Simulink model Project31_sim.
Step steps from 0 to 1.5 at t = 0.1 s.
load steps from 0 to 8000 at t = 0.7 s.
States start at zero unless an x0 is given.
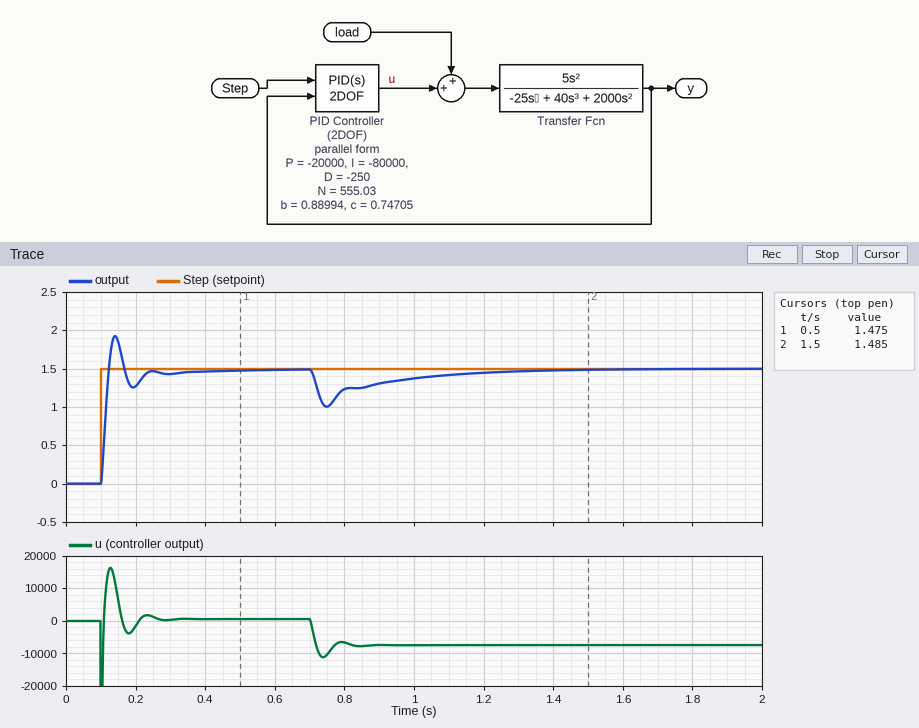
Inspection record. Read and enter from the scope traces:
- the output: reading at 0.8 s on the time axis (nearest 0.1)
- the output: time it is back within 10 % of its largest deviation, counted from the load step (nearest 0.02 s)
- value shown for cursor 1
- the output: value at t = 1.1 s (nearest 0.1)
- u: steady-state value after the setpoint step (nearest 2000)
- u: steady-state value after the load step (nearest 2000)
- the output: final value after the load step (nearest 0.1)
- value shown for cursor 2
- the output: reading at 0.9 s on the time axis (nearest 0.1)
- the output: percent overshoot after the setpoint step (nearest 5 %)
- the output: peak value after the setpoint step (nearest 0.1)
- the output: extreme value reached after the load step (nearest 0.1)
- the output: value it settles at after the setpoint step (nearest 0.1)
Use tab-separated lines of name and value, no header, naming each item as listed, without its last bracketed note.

the output: reading at 0.8 s on the time axis	1.2
the output: time it is back within 10 % of its largest deviation, counted from the load step	0.52 s
value shown for cursor 1	1.475
the output: value at t = 1.1 s	1.4
u: steady-state value after the setpoint step	0
u: steady-state value after the load step	-8000
the output: final value after the load step	1.5
value shown for cursor 2	1.485
the output: reading at 0.9 s on the time axis	1.3
the output: percent overshoot after the setpoint step	30 %
the output: peak value after the setpoint step	1.9
the output: extreme value reached after the load step	1.0
the output: value it settles at after the setpoint step	1.5
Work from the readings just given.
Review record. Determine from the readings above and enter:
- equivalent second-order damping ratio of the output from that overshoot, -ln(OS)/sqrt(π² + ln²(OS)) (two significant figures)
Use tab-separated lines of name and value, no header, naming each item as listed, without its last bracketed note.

equivalent second-order damping ratio of the output from that overshoot, -ln(OS)/sqrt(π² + ln²(OS))	0.36
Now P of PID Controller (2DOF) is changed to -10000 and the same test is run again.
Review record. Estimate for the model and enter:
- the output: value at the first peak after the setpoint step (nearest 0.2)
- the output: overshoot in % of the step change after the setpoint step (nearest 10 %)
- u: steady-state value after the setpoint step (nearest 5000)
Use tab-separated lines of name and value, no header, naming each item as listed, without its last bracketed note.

the output: value at the first peak after the setpoint step	1.8
the output: overshoot in % of the step change after the setpoint step	20 %
u: steady-state value after the setpoint step	0
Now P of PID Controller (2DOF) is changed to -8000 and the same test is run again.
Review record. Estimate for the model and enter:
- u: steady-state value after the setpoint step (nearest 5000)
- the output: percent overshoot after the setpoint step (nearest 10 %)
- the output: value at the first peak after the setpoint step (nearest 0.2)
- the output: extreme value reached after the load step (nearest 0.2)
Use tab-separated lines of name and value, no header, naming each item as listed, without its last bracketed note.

u: steady-state value after the setpoint step	0
the output: percent overshoot after the setpoint step	20 %
the output: value at the first peak after the setpoint step	1.8
the output: extreme value reached after the load step	0.6
